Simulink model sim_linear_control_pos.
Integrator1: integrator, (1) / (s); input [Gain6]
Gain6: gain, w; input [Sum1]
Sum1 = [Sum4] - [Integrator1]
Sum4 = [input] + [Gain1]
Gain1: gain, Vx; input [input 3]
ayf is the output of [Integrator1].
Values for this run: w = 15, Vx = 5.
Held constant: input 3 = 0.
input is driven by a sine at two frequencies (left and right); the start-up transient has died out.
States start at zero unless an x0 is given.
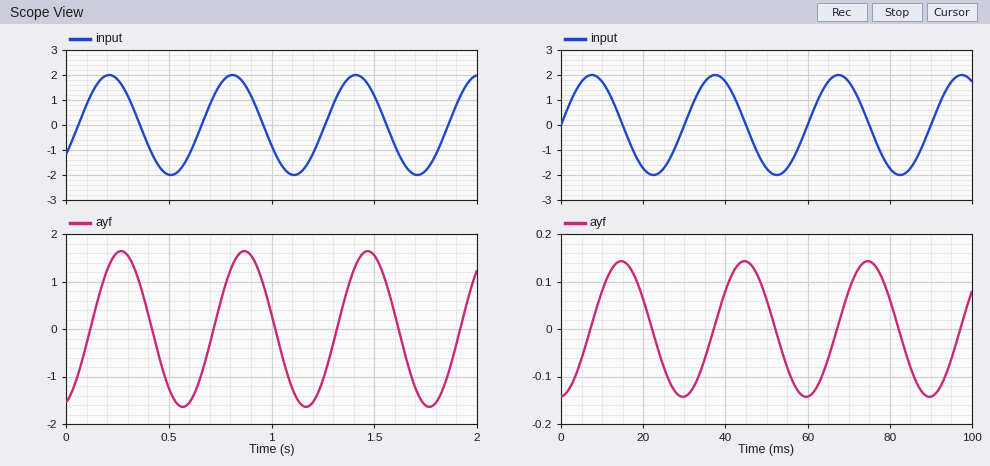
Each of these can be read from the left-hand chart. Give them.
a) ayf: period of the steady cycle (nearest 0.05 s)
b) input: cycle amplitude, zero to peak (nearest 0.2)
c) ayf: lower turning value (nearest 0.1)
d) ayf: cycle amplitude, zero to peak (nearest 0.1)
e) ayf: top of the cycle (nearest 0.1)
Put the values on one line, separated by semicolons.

0.60 s; 2.0; -1.6; 1.6; 1.6
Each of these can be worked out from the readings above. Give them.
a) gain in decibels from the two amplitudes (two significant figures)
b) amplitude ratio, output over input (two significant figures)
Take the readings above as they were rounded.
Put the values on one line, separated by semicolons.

-1.9 dB; 0.80
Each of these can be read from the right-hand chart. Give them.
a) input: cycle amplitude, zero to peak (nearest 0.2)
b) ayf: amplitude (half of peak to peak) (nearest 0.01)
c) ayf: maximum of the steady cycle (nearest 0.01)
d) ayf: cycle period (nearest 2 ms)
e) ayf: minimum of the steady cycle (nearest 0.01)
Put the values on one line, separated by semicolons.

2.0; 0.14; 0.14; 30 ms; -0.14
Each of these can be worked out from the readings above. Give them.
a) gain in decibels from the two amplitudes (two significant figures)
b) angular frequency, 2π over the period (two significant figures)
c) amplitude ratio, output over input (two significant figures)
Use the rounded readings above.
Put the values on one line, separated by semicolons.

-23 dB; 0.21 rad/ms; 0.070
